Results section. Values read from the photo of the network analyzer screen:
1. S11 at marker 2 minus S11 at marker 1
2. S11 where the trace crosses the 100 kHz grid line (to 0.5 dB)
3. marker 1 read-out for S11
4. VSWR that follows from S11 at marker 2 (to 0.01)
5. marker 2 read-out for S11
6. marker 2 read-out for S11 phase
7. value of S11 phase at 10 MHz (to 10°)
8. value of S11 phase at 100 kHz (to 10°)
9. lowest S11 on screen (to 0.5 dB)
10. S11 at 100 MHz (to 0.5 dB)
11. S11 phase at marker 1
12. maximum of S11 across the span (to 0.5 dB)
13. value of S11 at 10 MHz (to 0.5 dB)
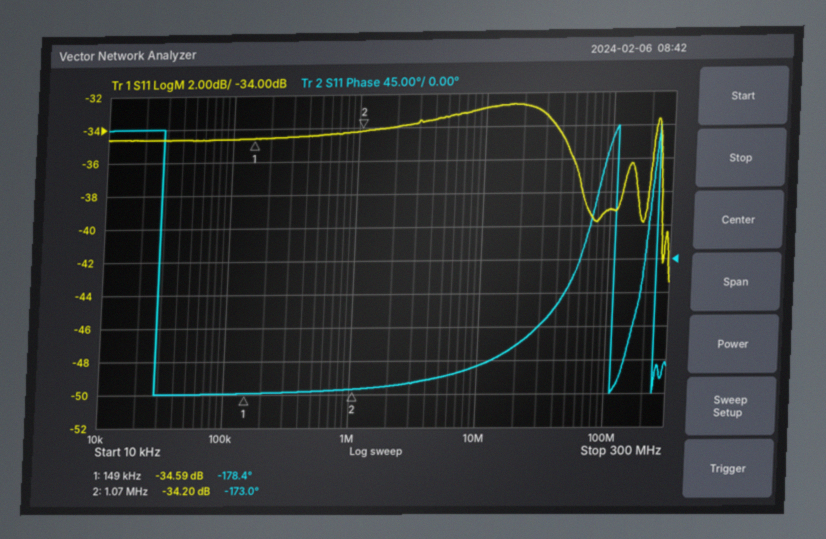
0.39 dB
-34.5 dB
-34.59 dB
1.04
-34.20 dB
-173.0°
-140°
-180°
-43.5 dB
-39.0 dB
-178.4°
-32.5 dB
-33.0 dB
